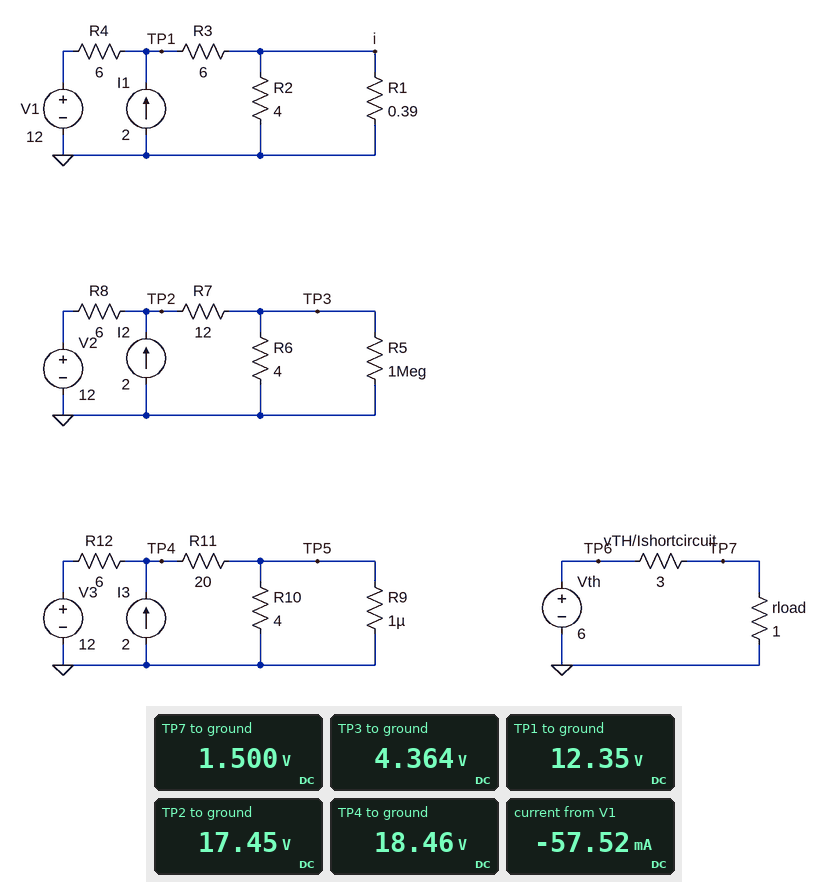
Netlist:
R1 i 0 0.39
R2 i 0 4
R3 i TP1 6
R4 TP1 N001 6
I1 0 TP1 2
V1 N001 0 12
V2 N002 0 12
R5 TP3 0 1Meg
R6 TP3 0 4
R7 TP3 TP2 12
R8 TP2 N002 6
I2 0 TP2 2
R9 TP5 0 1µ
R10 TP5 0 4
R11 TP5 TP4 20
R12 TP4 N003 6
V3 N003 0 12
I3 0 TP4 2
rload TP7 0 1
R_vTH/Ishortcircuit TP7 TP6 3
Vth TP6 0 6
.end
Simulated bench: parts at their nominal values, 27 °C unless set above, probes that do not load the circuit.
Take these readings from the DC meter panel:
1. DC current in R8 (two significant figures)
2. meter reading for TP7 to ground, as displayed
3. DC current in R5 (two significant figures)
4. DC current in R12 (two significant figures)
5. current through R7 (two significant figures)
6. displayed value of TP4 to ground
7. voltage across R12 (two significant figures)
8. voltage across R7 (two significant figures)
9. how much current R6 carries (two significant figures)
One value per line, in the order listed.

910 mA
1.500 V
4.4 µA
1.1 A
1.1 A
18.46 V
6.5 V
13 V
1.1 A
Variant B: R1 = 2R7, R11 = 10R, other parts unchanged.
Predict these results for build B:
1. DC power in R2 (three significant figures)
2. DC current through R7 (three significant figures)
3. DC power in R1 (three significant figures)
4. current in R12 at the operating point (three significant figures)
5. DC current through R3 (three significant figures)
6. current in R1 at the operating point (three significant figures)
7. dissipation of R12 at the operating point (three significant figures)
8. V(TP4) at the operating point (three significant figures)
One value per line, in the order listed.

2.02 W
1.09 A
2.99 W
500 mA
1.76 A
1.05 A
1.50 W
15.0 V
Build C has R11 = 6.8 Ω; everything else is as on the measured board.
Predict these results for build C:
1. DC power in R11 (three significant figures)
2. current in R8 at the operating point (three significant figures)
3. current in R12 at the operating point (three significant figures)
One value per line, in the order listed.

23.9 W
909 mA
125 mA
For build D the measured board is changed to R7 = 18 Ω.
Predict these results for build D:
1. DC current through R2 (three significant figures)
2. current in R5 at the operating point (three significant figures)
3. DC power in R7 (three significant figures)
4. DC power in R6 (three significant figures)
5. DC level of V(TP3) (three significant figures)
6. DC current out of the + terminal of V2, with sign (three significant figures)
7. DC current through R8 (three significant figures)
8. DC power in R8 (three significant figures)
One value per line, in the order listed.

173 mA
3.43 µA
13.2 W
2.94 W
3.43 V
-1.14 A
1.14 A
7.84 W
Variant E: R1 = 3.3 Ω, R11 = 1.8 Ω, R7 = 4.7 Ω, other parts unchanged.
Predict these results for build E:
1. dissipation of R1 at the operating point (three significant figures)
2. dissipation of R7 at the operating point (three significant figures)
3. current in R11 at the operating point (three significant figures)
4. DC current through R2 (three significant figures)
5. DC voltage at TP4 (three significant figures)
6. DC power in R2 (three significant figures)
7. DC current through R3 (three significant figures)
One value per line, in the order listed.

2.99 W
12.5 W
3.08 A
786 mA
5.54 V
2.47 W
1.74 A
